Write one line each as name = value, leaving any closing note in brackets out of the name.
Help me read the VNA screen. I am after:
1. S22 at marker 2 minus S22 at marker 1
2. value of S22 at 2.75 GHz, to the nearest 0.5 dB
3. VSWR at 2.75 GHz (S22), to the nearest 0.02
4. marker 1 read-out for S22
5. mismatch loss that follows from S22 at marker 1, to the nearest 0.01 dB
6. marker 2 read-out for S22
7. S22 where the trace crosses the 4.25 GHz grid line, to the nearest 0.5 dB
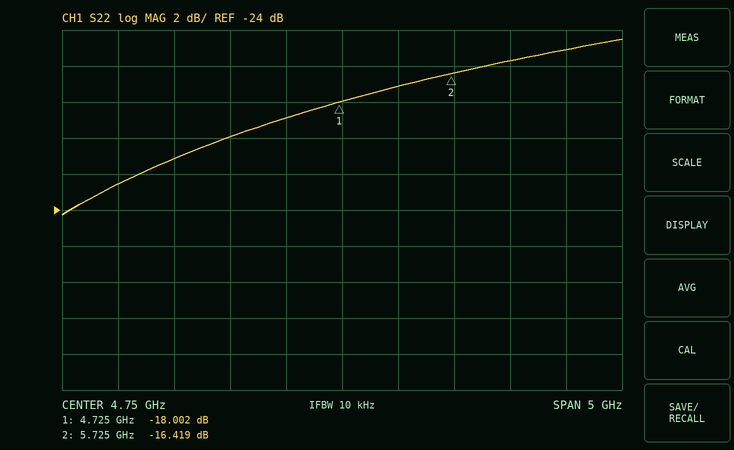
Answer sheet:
S22 at marker 2 minus S22 at marker 1 = 1.583 dB
value of S22 at 2.75 GHz, to the nearest 0.5 dB = -22.5 dB
VSWR at 2.75 GHz (S22), to the nearest 0.02 = 1.16
marker 1 read-out for S22 = -18.002 dB
mismatch loss that follows from S22 at marker 1, to the nearest 0.01 dB = 0.07 dB
marker 2 read-out for S22 = -16.419 dB
S22 where the trace crosses the 4.25 GHz grid line, to the nearest 0.5 dB = -19.0 dB
